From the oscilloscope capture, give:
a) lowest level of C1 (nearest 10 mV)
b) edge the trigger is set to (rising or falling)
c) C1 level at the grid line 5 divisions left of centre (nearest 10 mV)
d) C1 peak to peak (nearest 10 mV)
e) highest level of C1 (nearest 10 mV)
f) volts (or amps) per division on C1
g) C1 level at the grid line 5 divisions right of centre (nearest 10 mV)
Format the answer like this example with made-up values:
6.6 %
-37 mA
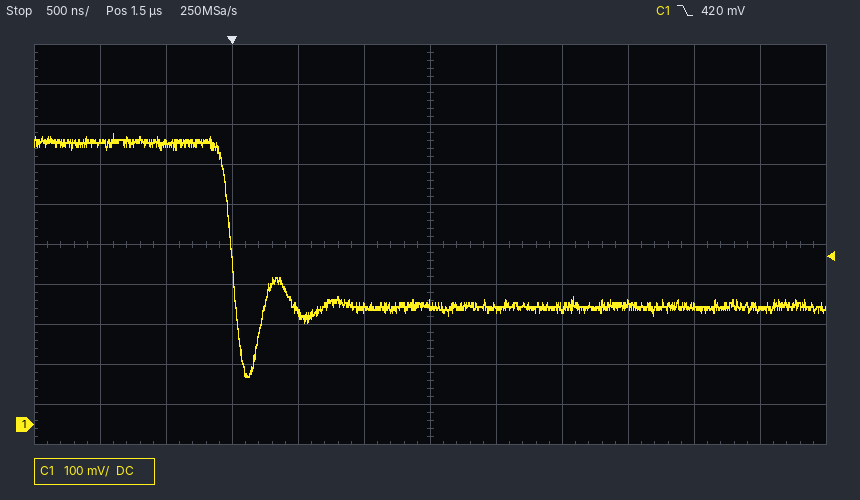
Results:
120 mV
falling
700 mV
610 mV
730 mV
100 mV
290 mV
